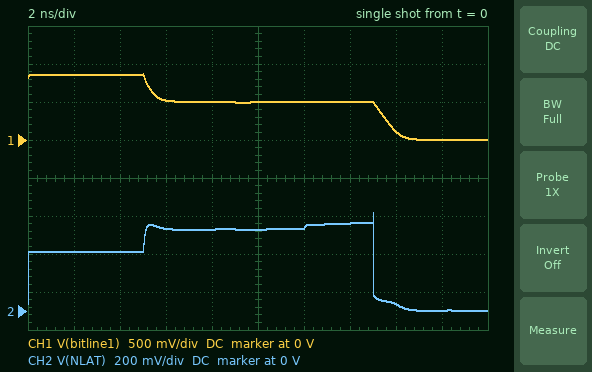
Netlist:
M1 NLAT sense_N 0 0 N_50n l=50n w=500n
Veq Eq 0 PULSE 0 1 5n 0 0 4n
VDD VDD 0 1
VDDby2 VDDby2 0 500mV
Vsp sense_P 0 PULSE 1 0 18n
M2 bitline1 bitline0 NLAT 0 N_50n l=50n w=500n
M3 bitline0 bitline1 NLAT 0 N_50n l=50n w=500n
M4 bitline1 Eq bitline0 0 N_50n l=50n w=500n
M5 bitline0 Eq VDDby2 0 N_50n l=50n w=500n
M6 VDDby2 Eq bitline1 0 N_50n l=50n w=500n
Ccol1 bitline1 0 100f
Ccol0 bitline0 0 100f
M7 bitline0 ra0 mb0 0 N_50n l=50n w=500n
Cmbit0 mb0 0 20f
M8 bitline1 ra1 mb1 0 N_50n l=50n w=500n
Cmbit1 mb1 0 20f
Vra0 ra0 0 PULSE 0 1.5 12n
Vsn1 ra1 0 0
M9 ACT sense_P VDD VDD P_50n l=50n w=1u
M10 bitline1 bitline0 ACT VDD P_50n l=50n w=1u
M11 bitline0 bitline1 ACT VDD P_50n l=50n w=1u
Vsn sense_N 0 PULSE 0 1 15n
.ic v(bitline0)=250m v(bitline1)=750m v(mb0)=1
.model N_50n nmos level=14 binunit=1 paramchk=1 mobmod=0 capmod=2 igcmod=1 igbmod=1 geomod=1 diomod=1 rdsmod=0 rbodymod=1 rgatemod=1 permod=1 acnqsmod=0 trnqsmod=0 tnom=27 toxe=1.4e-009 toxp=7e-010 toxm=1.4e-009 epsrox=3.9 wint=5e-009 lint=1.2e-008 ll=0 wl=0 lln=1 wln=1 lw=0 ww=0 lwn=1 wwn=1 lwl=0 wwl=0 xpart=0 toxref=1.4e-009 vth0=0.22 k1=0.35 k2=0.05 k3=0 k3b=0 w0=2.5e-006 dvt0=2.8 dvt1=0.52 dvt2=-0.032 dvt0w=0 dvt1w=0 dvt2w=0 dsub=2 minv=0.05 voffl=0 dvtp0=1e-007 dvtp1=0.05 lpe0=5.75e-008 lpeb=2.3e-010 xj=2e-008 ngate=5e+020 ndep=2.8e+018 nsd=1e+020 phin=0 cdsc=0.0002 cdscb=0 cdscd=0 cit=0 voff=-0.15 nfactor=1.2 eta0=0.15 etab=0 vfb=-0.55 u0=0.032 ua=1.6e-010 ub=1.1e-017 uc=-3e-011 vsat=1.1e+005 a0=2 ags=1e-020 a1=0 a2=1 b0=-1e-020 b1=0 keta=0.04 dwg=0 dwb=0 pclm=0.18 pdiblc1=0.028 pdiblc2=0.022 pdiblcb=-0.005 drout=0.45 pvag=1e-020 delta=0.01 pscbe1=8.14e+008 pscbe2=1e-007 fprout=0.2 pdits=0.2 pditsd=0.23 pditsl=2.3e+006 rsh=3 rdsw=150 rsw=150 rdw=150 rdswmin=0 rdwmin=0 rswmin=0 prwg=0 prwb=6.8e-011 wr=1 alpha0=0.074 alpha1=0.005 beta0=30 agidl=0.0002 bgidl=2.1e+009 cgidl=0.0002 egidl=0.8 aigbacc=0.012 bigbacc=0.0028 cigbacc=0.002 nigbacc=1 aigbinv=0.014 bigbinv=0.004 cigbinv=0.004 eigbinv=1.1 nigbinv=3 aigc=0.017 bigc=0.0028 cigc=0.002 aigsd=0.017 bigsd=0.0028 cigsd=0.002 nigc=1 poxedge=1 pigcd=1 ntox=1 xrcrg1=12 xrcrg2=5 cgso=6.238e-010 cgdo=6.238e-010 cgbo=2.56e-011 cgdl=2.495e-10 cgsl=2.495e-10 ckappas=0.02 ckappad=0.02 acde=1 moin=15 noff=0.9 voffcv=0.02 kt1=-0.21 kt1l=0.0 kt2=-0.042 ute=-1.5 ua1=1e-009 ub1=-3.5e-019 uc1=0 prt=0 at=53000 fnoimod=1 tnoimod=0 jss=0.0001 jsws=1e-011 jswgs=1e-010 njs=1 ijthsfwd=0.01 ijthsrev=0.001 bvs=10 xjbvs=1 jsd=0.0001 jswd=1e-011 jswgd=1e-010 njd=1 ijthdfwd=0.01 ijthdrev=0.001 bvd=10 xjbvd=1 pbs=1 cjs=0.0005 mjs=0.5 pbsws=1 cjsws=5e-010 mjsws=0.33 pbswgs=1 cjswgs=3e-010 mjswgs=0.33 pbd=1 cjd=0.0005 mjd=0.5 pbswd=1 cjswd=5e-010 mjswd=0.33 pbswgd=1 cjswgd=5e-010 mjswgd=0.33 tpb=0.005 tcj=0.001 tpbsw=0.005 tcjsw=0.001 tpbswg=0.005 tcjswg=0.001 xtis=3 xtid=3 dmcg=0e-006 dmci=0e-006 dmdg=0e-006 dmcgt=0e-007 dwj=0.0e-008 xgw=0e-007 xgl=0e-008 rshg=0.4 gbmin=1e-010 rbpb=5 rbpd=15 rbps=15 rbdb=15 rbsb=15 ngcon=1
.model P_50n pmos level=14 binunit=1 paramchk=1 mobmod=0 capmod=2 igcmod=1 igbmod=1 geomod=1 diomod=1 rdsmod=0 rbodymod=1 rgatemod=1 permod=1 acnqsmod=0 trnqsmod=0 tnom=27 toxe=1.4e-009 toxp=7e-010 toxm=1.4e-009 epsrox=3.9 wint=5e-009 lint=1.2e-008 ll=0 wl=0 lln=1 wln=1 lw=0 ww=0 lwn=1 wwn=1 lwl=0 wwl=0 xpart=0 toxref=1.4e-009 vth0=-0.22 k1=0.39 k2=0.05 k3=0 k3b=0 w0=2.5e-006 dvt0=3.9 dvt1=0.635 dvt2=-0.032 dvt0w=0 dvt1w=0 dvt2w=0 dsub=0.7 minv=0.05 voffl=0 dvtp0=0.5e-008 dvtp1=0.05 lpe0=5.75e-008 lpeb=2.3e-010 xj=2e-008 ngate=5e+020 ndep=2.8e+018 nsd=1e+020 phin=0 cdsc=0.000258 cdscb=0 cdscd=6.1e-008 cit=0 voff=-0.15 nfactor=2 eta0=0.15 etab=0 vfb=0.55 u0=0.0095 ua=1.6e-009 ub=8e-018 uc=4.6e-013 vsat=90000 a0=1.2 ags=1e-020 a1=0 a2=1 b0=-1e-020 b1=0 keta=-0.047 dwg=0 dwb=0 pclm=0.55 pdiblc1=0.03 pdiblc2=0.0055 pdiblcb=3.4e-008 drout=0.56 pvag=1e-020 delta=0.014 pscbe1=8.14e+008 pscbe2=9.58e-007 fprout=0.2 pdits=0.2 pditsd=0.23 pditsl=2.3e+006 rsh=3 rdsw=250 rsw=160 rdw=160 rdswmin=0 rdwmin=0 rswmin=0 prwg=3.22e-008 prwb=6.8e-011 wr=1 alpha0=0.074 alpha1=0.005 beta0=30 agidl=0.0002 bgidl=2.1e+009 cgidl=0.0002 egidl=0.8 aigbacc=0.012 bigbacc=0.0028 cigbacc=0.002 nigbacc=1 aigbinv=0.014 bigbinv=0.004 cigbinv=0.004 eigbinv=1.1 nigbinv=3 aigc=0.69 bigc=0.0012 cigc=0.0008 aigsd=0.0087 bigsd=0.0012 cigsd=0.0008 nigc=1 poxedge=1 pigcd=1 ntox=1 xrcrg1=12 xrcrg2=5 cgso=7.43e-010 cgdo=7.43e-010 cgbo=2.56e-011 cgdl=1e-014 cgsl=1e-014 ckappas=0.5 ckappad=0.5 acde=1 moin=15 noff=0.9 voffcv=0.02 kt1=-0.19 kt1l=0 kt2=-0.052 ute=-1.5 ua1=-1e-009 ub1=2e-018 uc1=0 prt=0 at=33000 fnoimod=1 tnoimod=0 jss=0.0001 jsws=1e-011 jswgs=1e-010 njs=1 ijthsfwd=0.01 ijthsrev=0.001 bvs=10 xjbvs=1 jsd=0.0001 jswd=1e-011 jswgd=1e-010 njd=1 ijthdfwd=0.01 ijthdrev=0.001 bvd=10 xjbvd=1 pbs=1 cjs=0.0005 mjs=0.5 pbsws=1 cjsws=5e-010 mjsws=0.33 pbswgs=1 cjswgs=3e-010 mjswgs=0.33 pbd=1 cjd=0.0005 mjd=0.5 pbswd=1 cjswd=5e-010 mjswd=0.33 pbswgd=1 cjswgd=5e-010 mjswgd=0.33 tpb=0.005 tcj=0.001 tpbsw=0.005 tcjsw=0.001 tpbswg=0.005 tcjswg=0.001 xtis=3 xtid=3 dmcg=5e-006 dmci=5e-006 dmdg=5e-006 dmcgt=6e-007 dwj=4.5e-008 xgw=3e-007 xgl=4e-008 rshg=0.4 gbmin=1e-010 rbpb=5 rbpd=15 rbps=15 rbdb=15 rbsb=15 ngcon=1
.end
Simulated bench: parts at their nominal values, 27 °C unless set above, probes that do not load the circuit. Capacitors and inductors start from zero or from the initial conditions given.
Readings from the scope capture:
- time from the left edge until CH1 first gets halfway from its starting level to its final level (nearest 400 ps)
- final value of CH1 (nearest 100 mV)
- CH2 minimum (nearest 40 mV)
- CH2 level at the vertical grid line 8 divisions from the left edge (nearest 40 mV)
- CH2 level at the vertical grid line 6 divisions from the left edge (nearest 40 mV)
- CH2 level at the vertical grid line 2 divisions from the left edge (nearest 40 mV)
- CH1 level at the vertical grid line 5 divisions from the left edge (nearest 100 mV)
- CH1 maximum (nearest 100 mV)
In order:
15.2 ns
0 V
0 V
40 mV
440 mV
320 mV
500 mV
900 mV
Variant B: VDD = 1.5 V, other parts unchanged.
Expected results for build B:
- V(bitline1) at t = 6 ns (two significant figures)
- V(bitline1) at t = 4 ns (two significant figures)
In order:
1.2 V
1.5 V
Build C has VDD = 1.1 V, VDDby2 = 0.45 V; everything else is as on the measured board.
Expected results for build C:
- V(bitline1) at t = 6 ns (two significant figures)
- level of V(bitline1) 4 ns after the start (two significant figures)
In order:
460 mV
890 mV
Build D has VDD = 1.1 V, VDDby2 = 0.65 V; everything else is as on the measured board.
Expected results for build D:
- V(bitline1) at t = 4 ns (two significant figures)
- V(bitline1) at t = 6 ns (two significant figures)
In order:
890 mV
730 mV
